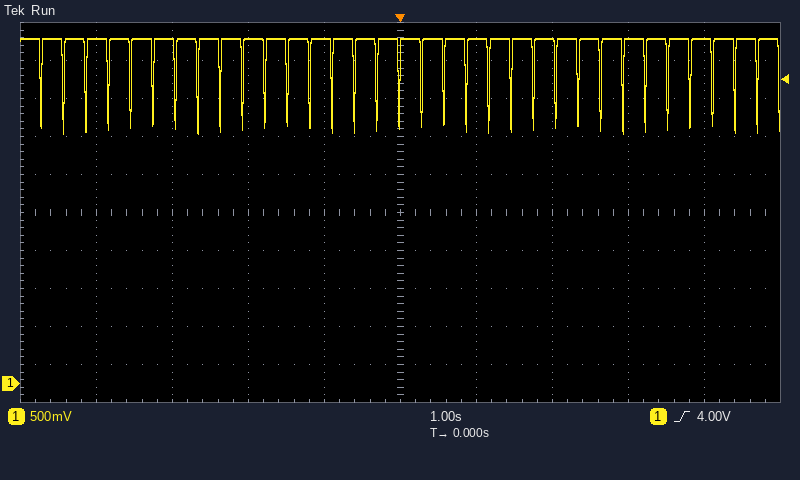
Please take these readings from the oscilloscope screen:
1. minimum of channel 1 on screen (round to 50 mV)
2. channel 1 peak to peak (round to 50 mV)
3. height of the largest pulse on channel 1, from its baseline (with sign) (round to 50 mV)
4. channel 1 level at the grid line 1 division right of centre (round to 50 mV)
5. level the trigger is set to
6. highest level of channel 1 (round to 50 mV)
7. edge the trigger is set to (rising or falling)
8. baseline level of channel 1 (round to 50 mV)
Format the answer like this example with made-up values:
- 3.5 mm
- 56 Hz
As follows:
- 3.30 V
- 1.25 V
- -1.25 V
- 4.55 V
- 4.00 V
- 4.55 V
- rising
- 4.55 V
